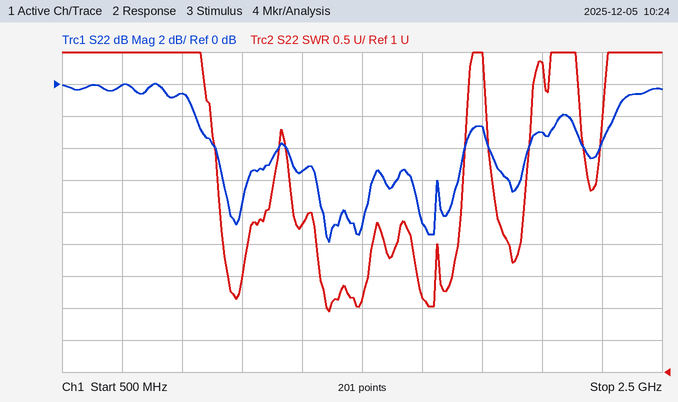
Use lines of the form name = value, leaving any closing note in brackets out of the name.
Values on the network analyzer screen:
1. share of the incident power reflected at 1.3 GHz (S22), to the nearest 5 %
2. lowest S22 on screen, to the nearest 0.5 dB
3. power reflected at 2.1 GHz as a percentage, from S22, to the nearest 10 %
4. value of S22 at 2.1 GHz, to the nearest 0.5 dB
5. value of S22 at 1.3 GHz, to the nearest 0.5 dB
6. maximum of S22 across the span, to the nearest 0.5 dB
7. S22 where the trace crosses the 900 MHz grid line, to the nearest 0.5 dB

share of the incident power reflected at 1.3 GHz (S22), to the nearest 5 % = 30 %
lowest S22 on screen, to the nearest 0.5 dB = -10.0 dB
power reflected at 2.1 GHz as a percentage, from S22, to the nearest 10 % = 50 %
value of S22 at 2.1 GHz, to the nearest 0.5 dB = -3.0 dB
value of S22 at 1.3 GHz, to the nearest 0.5 dB = -5.5 dB
maximum of S22 across the span, to the nearest 0.5 dB = 0.0 dB
S22 where the trace crosses the 900 MHz grid line, to the nearest 0.5 dB = -0.5 dB
